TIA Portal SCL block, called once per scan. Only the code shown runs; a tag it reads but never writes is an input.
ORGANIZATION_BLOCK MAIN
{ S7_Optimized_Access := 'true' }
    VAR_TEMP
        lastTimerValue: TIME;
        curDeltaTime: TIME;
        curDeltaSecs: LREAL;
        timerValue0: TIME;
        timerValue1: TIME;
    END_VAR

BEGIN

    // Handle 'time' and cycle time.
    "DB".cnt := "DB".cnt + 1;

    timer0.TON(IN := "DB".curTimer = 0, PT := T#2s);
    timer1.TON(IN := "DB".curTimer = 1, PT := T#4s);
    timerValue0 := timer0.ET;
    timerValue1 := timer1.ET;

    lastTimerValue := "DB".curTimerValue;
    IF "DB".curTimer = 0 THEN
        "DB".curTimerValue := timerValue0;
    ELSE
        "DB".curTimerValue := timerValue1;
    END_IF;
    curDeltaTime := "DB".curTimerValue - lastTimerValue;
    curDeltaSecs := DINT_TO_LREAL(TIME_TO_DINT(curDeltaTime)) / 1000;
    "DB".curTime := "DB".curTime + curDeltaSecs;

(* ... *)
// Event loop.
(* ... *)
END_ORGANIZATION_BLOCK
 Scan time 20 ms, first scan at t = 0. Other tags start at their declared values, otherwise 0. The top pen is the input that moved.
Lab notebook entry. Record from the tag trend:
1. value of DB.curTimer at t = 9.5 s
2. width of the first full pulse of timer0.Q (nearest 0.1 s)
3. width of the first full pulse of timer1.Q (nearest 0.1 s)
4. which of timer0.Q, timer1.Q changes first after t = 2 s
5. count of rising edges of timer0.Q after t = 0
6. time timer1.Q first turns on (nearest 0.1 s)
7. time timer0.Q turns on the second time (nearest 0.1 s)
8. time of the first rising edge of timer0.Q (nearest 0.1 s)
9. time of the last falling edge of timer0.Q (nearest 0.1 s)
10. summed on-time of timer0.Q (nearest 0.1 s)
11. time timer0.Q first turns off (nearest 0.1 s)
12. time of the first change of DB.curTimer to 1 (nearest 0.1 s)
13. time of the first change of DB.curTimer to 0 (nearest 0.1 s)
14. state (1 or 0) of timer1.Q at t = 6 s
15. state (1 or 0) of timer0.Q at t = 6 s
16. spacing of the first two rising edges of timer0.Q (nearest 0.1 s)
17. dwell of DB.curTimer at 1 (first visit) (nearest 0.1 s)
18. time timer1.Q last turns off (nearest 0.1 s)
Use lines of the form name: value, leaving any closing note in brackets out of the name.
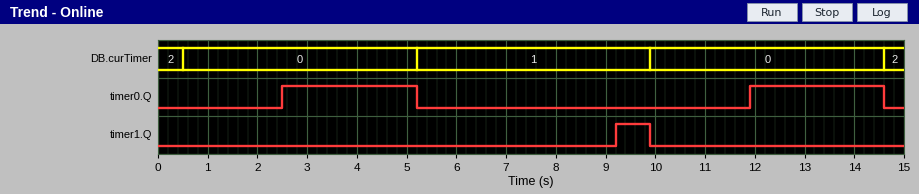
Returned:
value of DB.curTimer at t = 9.5 s: 1
width of the first full pulse of timer0.Q: 2.7 s
width of the first full pulse of timer1.Q: 0.7 s
which of timer0.Q, timer1.Q changes first after t = 2 s: timer0.Q
count of rising edges of timer0.Q after t = 0: 2
time timer1.Q first turns on: 9.2 s
time timer0.Q turns on the second time: 11.9 s
time of the first rising edge of timer0.Q: 2.5 s
time of the last falling edge of timer0.Q: 14.6 s
summed on-time of timer0.Q: 5.4 s
time timer0.Q first turns off: 5.2 s
time of the first change of DB.curTimer to 1: 5.2 s
time of the first change of DB.curTimer to 0: 0.5 s
state (1 or 0) of timer1.Q at t = 6 s: 0
state (1 or 0) of timer0.Q at t = 6 s: 0
spacing of the first two rising edges of timer0.Q: 9.4 s
dwell of DB.curTimer at 1 (first visit): 4.7 s
time timer1.Q last turns off: 9.9 s
